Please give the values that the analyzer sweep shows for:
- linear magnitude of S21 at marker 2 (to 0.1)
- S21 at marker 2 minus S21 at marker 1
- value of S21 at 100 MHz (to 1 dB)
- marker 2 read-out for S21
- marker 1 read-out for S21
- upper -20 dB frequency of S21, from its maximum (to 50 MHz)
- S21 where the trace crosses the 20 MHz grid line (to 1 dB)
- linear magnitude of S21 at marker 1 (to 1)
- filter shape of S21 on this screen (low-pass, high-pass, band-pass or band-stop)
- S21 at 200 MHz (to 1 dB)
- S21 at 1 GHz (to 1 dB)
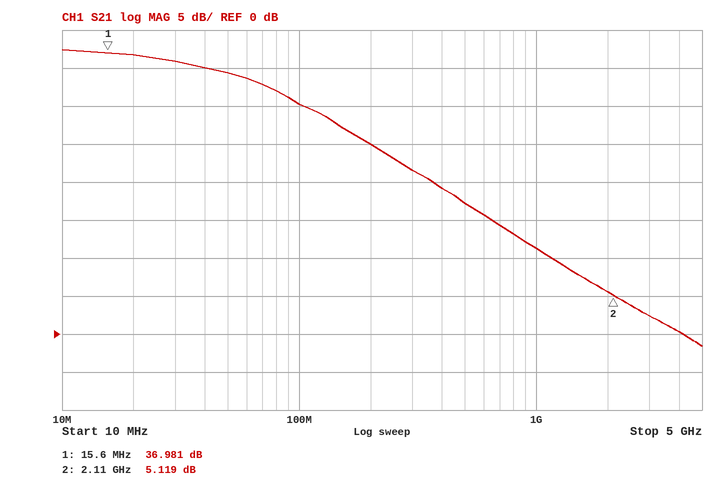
1.8
-31.862 dB
30 dB
5.119 dB
36.981 dB
500 MHz
37 dB
71
low-pass
25 dB
11 dB
